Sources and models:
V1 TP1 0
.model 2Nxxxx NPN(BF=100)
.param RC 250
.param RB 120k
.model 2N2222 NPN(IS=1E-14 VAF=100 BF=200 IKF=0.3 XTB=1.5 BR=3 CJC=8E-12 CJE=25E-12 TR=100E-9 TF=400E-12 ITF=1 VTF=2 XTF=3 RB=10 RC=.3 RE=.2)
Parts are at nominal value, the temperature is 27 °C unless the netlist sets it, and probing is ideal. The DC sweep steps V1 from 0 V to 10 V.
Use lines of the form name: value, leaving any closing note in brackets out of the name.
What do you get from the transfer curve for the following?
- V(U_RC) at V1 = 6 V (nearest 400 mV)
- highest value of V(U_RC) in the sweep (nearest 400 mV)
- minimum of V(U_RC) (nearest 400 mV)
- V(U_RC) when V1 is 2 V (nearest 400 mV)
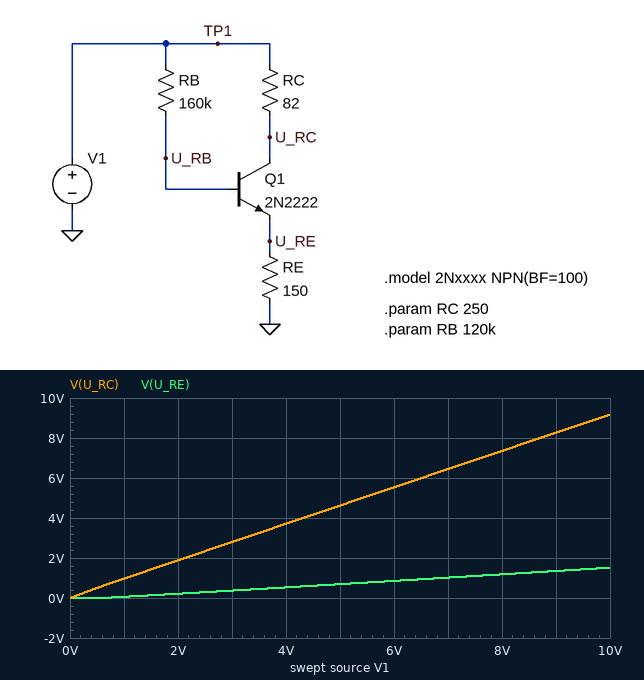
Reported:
V(U_RC) at V1 = 6 V: 5.6 V
highest value of V(U_RC) in the sweep: 9.2 V
minimum of V(U_RC): 0 V
V(U_RC) when V1 is 2 V: 2.0 V
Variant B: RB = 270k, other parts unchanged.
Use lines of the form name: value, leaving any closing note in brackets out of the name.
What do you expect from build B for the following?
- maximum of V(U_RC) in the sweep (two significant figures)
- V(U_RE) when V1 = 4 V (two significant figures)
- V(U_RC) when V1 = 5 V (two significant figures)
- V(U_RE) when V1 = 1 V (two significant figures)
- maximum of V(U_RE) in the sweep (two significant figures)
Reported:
maximum of V(U_RC) in the sweep: 9.5 V
V(U_RE) when V1 = 4 V: 340 mV
V(U_RC) when V1 = 5 V: 4.8 V
V(U_RE) when V1 = 1 V: 38 mV
maximum of V(U_RE) in the sweep: 980 mV
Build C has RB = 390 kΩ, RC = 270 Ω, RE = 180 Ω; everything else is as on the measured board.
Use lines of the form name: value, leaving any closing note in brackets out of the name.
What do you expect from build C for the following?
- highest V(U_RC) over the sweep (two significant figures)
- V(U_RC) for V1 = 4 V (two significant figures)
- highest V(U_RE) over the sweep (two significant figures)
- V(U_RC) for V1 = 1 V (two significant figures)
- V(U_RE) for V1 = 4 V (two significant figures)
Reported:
highest V(U_RC) over the sweep: 8.8 V
V(U_RC) for V1 = 4 V: 3.6 V
highest V(U_RE) over the sweep: 830 mV
V(U_RC) for V1 = 1 V: 950 mV
V(U_RE) for V1 = 4 V: 290 mV
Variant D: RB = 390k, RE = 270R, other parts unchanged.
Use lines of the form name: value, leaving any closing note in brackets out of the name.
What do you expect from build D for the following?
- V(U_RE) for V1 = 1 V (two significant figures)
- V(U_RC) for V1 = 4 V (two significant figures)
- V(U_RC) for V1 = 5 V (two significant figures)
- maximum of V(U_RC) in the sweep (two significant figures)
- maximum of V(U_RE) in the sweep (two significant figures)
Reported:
V(U_RE) for V1 = 1 V: 48 mV
V(U_RC) for V1 = 4 V: 3.9 V
V(U_RC) for V1 = 5 V: 4.8 V
maximum of V(U_RC) in the sweep: 9.6 V
maximum of V(U_RE) in the sweep: 1.2 V
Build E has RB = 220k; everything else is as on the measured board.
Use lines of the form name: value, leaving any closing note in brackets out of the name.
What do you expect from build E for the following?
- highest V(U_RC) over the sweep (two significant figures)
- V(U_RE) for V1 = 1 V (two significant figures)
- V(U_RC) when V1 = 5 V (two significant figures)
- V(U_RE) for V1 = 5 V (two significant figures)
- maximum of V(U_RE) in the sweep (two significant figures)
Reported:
highest V(U_RC) over the sweep: 9.4 V
V(U_RE) for V1 = 1 V: 45 mV
V(U_RC) when V1 = 5 V: 4.7 V
V(U_RE) for V1 = 5 V: 530 mV
maximum of V(U_RE) in the sweep: 1.2 V
